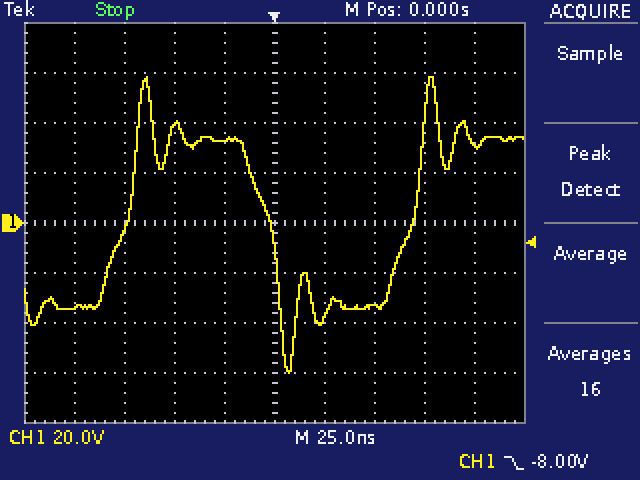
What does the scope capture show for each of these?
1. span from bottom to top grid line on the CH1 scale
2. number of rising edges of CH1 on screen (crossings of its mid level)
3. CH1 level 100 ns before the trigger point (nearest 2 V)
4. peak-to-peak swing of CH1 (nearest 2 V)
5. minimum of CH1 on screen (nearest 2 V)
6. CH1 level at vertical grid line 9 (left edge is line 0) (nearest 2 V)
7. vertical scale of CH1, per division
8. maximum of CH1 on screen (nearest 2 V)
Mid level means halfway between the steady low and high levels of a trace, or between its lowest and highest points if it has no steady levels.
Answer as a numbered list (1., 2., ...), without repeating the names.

1. 160 V
2. 2
3. -34 V
4. 118 V
5. -60 V
6. 32 V
7. 20 V
8. 58 V
